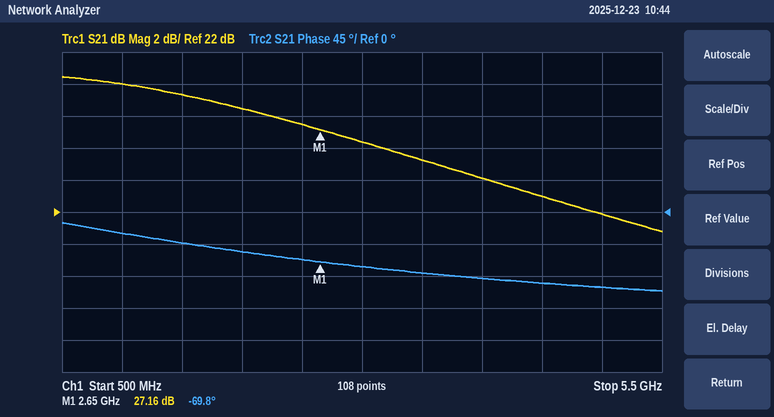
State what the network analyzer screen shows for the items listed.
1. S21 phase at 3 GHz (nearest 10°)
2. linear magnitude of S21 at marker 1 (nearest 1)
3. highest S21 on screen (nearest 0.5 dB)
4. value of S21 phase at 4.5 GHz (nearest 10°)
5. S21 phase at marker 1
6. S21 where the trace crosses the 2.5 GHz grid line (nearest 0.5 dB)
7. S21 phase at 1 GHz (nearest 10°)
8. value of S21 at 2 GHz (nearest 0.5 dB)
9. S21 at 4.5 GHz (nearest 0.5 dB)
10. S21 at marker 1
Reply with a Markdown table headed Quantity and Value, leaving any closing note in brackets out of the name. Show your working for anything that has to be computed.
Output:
| Quantity | Value |
|---|---|
| S21 phase at 3 GHz | -80° |
| linear magnitude of S21 at marker 1 | 10^(27.16/20) ≈ 23 |
| highest S21 on screen | 30.5 dB |
| value of S21 phase at 4.5 GHz | -100° |
| S21 phase at marker 1 | -69.8° |
| S21 where the trace crosses the 2.5 GHz grid line | 27.5 dB |
| S21 phase at 1 GHz | -30° |
| value of S21 at 2 GHz | 28.5 dB |
| S21 at 4.5 GHz | 23.0 dB |
| S21 at marker 1 | 27.16 dB |
